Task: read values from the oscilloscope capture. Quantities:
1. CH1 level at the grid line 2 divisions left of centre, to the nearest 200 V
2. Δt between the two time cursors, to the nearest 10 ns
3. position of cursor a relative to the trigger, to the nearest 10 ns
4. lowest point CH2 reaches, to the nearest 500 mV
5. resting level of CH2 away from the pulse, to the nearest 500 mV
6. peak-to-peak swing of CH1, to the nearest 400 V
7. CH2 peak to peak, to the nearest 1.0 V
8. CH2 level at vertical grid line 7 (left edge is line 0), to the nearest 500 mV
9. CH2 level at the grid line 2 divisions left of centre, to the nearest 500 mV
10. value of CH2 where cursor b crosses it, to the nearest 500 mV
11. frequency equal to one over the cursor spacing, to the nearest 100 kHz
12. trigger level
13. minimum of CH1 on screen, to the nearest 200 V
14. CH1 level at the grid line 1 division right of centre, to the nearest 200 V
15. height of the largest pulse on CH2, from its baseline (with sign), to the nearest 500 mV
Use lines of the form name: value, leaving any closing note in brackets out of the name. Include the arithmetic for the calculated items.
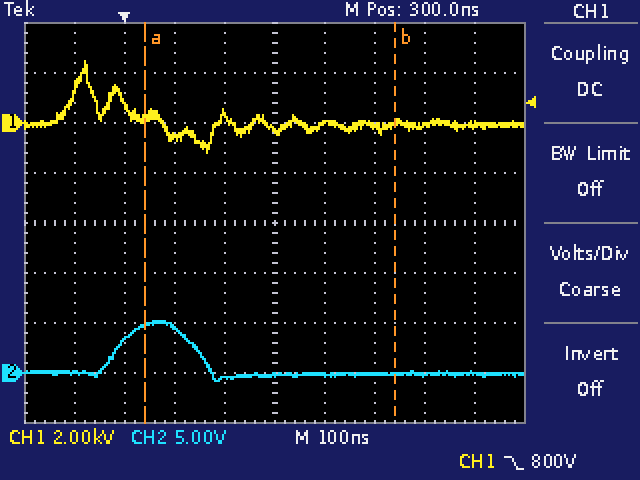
CH1 level at the grid line 2 divisions left of centre, to the nearest 200 V: -600 V
Δt between the two time cursors, to the nearest 10 ns: 500 ns
position of cursor a relative to the trigger, to the nearest 10 ns: +40 ns
lowest point CH2 reaches, to the nearest 500 mV: -1.0 V
resting level of CH2 away from the pulse, to the nearest 500 mV: 0.0 V
peak-to-peak swing of CH1, to the nearest 400 V: 3.6 kV
CH2 peak to peak, to the nearest 1.0 V: 6.0 V
CH2 level at vertical grid line 7 (left edge is line 0), to the nearest 500 mV: 0.0 V
CH2 level at the grid line 2 divisions left of centre, to the nearest 500 mV: 4.5 V
value of CH2 where cursor b crosses it, to the nearest 500 mV: 0.0 V
frequency equal to one over the cursor spacing, to the nearest 100 kHz: 1 / 500 ns ≈ 2.0 MHz
trigger level: 800 V
minimum of CH1 on screen, to the nearest 200 V: -1.2 kV
CH1 level at the grid line 1 division right of centre, to the nearest 200 V: 0.0 kV
height of the largest pulse on CH2, from its baseline (with sign), to the nearest 500 mV: +5.5 V
